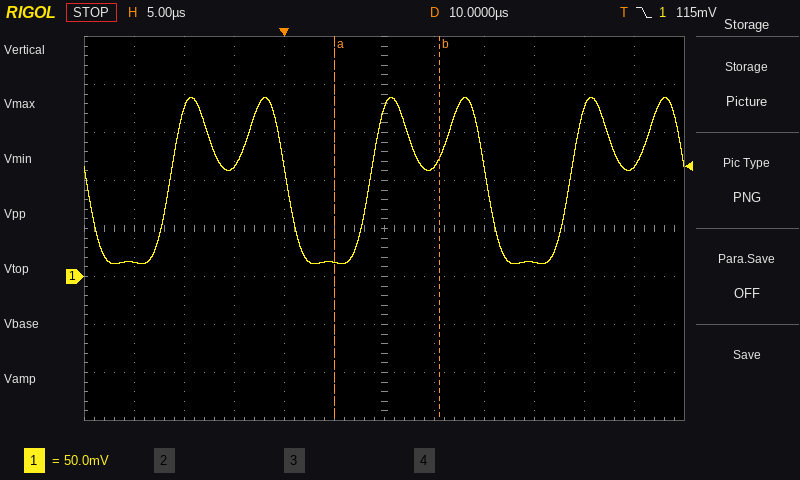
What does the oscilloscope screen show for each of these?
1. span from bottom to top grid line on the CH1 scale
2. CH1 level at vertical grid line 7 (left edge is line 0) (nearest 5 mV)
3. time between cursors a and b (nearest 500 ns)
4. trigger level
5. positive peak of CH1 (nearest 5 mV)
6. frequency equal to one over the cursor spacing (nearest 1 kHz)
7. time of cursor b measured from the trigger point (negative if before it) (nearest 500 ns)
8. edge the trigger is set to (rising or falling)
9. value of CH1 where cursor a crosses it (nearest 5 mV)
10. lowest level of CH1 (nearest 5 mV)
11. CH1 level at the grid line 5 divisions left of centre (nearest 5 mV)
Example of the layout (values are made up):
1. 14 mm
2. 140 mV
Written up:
1. 400 mV
2. 115 mV
3. 10.5 µs
4. 115 mV
5. 185 mV
6. 95 kHz
7. +15.5 µs
8. falling
9. 15 mV
10. 15 mV
11. 15 mV
